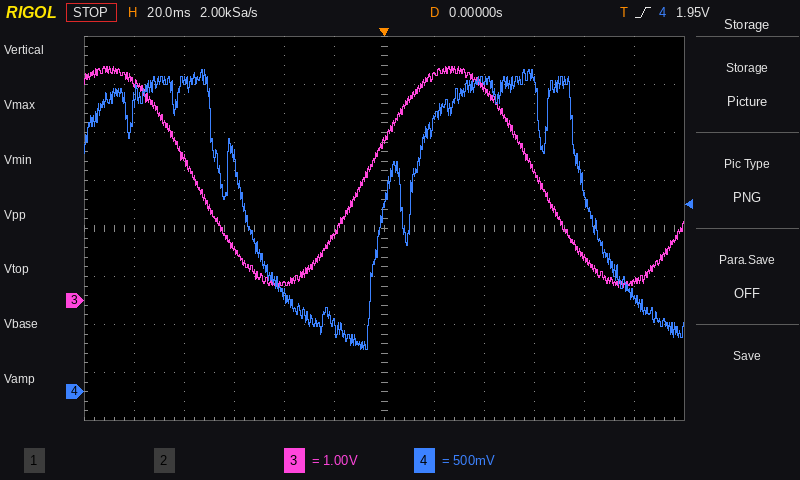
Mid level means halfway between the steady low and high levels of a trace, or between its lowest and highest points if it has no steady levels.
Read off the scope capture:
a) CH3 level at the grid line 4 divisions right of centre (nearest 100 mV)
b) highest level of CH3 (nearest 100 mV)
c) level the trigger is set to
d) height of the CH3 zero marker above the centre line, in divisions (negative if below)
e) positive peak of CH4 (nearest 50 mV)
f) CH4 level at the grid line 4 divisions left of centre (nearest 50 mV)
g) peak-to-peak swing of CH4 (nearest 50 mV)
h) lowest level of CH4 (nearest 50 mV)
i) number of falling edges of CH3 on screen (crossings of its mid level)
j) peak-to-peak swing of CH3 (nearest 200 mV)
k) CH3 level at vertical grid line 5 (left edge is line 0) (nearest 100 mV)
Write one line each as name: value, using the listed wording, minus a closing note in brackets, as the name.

CH3 level at the grid line 4 divisions right of centre: 900 mV
highest level of CH3: 4.9 V
level the trigger is set to: 1.95 V
height of the CH3 zero marker above the centre line, in divisions: -1.5 div
positive peak of CH4: 3.35 V
CH4 level at the grid line 4 divisions left of centre: 3.25 V
peak-to-peak swing of CH4: 2.90 V
lowest level of CH4: 450 mV
number of falling edges of CH3 on screen: 2
peak-to-peak swing of CH3: 4.6 V
CH3 level at vertical grid line 5 (left edge is line 0): 1.4 V
